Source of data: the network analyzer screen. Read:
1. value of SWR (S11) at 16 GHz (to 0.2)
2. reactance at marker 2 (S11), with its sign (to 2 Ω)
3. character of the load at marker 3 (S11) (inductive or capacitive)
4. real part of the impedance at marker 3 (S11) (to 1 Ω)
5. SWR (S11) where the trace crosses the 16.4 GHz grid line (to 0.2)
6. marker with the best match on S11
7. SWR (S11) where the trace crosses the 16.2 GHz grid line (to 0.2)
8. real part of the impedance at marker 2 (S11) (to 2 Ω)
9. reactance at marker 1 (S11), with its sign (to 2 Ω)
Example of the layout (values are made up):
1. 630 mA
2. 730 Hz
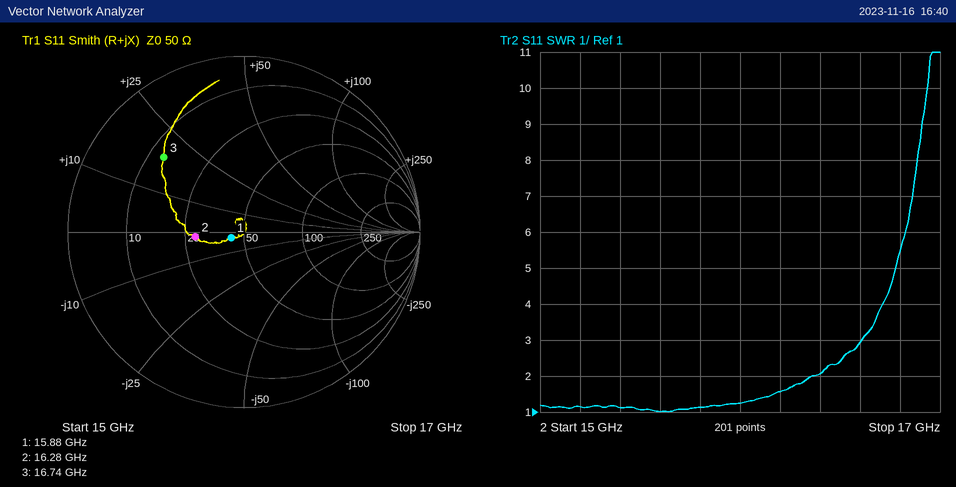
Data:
1. 1.2
2. -2 Ω
3. inductive
4. 13 Ω
5. 2.0
6. marker 1
7. 1.6
8. 28 Ω
9. -2 Ω
